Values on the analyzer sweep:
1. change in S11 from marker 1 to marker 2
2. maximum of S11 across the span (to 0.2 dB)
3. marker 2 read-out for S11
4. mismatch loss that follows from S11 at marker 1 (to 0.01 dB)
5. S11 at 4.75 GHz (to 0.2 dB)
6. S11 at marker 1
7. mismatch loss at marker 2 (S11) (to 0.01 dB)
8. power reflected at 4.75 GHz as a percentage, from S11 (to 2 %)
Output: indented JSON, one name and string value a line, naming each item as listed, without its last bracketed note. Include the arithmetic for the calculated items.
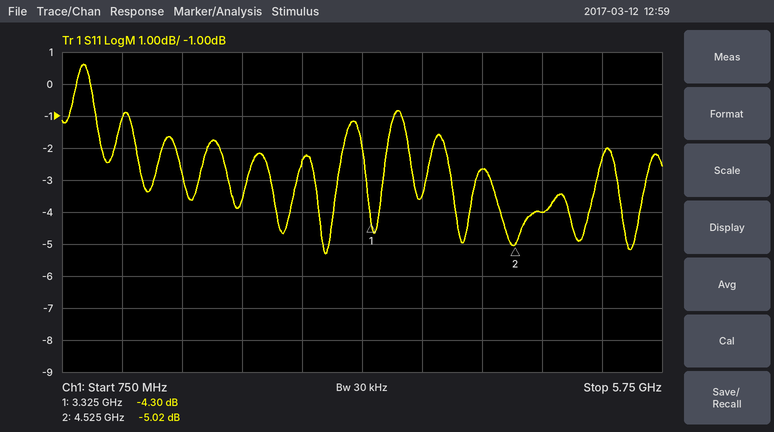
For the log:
{
  "change in S11 from marker 1 to marker 2": "-5.02 − (-4.3) = -0.72 dB",
  "maximum of S11 across the span": "0.6 dB",
  "marker 2 read-out for S11": "-5.02 dB",
  "mismatch loss that follows from S11 at marker 1": "−10 log10(1 − 10^(-4.3/10)) ≈ 2.02 dB",
  "S11 at 4.75 GHz": "-4.0 dB",
  "S11 at marker 1": "-4.30 dB",
  "mismatch loss at marker 2 (S11)": "−10 log10(1 − 10^(-5.02/10)) ≈ 1.64 dB",
  "power reflected at 4.75 GHz as a percentage, from S11": "10^(-4/10) ≈ 40 %"
}
